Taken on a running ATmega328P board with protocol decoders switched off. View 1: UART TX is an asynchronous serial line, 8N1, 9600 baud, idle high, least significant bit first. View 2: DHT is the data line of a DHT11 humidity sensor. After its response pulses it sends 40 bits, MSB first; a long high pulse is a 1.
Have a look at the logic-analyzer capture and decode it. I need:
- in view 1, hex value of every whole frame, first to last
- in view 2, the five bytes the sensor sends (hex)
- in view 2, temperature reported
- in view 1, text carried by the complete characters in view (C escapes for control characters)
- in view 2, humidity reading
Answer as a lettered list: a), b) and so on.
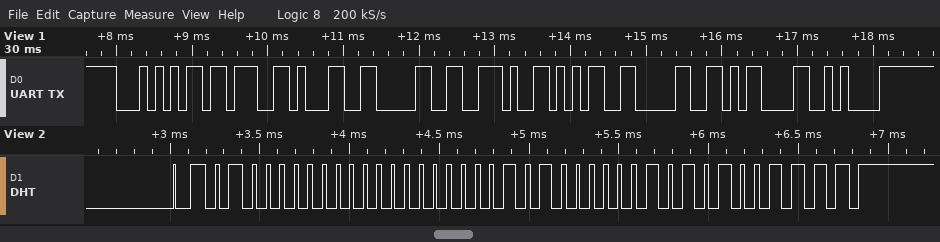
a) 54 3B 31 30 2E 35 30 0D 0A
b) 40 00 0A 05 4F
c) 10.5 °C
d) "T;10.50\r\n"
e) 64 %
